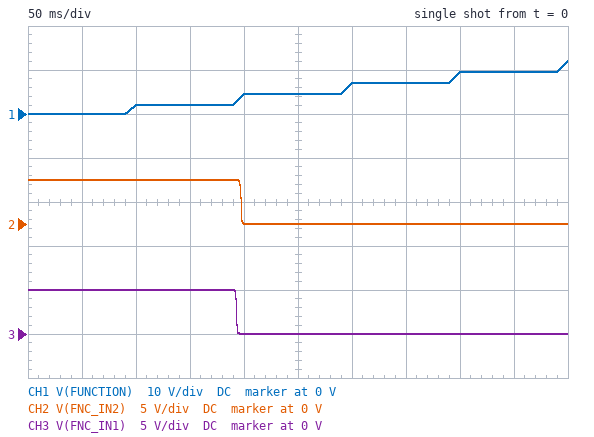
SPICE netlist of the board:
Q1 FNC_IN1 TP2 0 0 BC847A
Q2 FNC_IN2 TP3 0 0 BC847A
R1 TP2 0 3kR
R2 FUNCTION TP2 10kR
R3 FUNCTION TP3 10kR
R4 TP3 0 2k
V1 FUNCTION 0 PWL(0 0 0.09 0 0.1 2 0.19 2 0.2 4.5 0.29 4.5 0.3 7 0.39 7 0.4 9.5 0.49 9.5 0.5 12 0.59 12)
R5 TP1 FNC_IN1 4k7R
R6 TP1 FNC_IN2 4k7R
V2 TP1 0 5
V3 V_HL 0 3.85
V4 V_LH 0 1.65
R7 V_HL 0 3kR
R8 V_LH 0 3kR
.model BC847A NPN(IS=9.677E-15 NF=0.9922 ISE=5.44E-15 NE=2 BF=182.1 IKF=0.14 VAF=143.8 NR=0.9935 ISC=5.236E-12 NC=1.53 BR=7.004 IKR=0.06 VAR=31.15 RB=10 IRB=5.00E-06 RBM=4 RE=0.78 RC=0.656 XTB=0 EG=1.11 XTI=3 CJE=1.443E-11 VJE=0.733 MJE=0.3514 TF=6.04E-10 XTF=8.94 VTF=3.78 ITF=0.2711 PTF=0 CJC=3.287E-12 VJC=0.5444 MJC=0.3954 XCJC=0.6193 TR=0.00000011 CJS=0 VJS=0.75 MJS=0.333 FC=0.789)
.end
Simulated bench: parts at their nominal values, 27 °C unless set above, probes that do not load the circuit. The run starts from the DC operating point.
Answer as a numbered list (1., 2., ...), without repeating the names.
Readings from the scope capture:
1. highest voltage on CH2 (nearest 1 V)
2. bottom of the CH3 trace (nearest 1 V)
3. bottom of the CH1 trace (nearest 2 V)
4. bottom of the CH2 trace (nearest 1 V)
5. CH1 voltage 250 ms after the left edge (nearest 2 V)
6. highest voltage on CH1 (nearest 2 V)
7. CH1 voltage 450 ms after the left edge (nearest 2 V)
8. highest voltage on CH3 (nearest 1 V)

1. 5 V
2. 0 V
3. 0 V
4. 0 V
5. 4 V
6. 12 V
7. 10 V
8. 5 V
